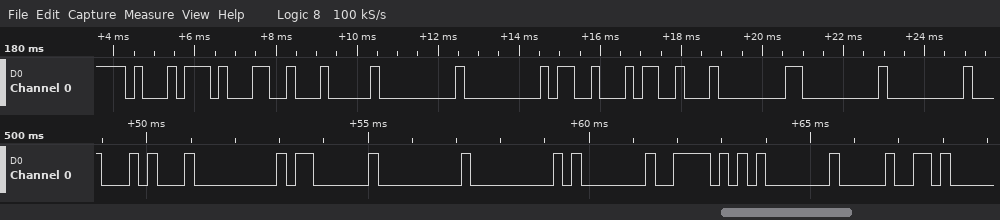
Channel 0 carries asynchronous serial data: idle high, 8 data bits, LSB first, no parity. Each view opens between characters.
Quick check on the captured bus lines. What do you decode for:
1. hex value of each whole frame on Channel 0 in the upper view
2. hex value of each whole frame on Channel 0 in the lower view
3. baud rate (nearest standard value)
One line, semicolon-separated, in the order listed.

D1, 31, 04, 00, 00, 13, 13, 80, 00, 00; 14, 00, 03, 00, 00, 01, 5E, 01, 90; 4800 baud
